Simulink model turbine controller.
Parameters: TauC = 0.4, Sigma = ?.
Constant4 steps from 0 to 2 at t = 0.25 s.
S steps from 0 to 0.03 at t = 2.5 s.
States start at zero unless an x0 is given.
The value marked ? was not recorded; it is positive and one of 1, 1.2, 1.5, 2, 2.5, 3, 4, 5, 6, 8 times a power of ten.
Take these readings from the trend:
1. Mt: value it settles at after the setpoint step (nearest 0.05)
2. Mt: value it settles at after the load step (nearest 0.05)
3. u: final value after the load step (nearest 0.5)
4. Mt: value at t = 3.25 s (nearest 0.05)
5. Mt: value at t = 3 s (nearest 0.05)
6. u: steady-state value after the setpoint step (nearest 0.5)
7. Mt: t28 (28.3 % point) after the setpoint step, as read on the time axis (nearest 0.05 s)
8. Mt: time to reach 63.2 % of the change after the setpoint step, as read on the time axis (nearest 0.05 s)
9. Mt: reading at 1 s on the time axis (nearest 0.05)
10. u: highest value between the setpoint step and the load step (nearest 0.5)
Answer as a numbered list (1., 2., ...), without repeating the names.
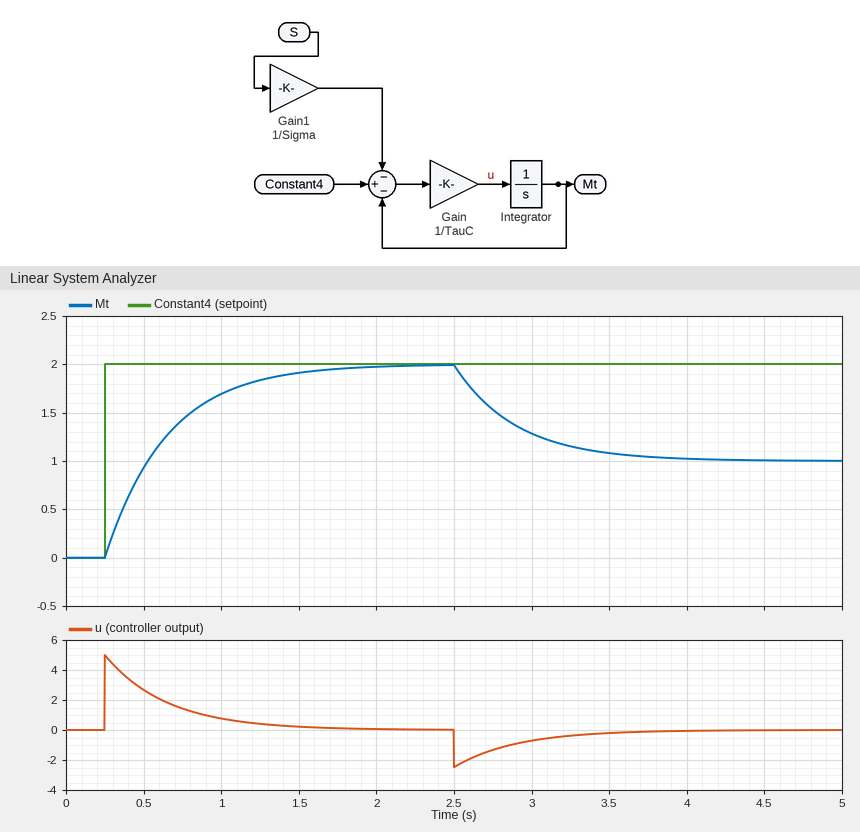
1. 2.00
2. 1.00
3. 0.0
4. 1.15
5. 1.30
6. 0.0
7. 0.40 s
8. 0.65 s
9. 1.70
10. 5.0
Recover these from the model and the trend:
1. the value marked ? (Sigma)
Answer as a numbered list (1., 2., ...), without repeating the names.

1. 0.03
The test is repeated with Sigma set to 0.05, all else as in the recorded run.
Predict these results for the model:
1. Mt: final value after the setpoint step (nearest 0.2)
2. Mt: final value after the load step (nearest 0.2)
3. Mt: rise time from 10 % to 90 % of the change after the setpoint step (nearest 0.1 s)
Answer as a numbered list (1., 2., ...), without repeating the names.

1. 2.0
2. 1.4
3. 0.9 s
